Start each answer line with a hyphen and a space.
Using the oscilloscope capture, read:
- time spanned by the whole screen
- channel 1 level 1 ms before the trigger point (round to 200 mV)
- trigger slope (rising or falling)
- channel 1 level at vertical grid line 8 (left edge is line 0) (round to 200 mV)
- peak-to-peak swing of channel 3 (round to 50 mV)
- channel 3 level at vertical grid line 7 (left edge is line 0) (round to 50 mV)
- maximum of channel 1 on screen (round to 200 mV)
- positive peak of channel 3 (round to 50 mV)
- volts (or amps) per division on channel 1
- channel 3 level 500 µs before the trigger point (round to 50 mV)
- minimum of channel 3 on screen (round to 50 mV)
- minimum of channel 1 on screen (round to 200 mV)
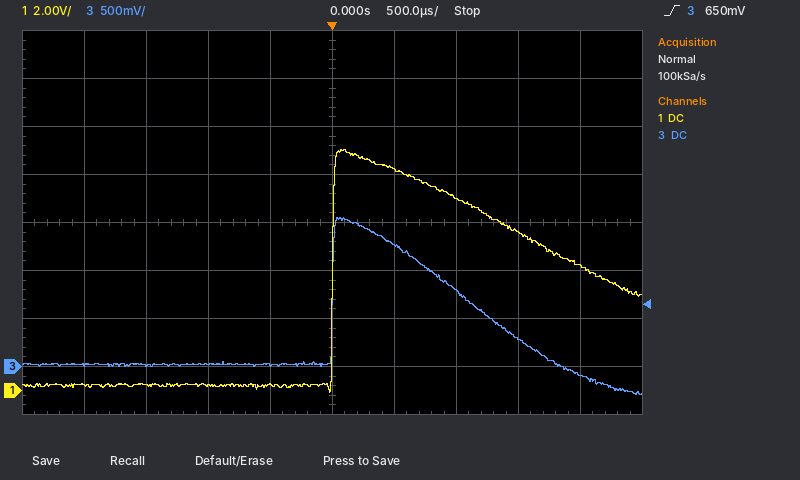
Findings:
- 5 ms
- 200 mV
- rising
- 6.6 V
- 1.85 V
- 800 mV
- 10.0 V
- 1.55 V
- 2 V
- 0 mV
- -300 mV
- 0.0 V
